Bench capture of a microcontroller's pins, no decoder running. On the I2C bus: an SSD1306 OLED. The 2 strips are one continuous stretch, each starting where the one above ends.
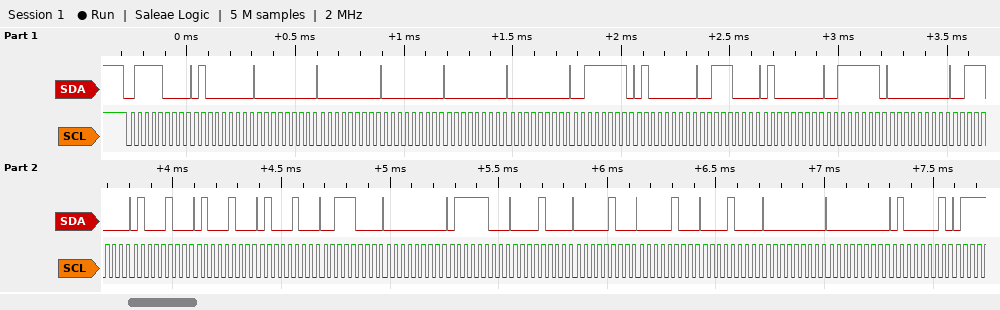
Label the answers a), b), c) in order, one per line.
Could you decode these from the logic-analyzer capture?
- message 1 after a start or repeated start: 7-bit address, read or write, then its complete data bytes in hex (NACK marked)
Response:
a) 0x3C write: 40 00 00 00 00 00 3F 40 38 40 3F 00 38 44 44 44 38 00 7C 08 04 04 08 00 00 41
